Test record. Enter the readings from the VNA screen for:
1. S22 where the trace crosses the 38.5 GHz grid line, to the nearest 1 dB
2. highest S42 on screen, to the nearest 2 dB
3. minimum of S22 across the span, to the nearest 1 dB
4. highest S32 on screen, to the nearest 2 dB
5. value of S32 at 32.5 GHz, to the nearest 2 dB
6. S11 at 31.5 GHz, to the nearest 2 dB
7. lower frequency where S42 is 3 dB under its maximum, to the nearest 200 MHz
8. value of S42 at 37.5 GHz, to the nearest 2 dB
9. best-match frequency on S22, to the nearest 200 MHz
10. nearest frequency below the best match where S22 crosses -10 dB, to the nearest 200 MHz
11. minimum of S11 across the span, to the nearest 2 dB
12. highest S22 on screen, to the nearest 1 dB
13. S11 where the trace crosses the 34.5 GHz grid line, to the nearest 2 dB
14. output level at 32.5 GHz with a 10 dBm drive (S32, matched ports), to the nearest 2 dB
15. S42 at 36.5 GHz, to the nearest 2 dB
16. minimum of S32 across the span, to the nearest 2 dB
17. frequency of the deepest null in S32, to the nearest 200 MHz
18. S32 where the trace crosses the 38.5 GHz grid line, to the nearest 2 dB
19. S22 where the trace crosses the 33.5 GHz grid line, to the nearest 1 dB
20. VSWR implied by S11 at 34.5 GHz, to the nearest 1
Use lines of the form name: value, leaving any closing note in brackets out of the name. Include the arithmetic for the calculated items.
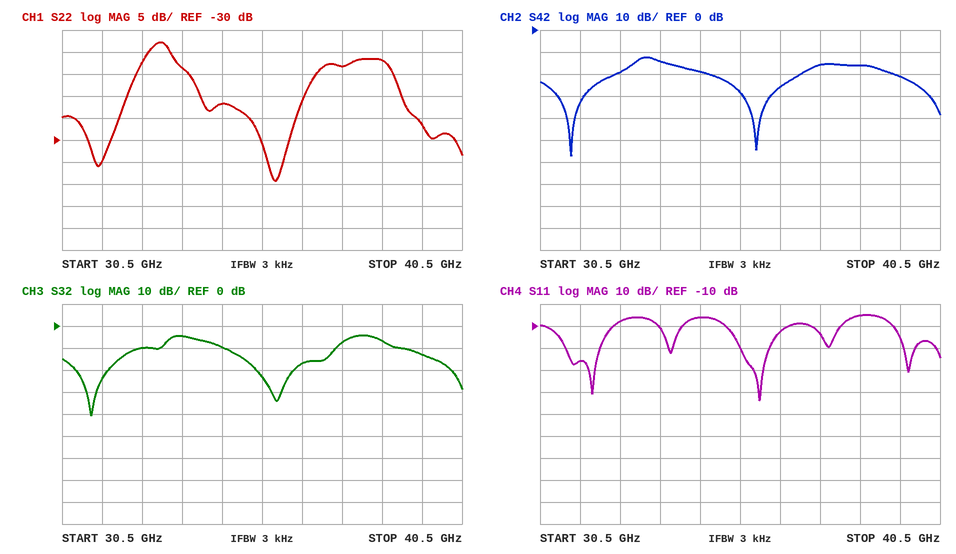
S22 where the trace crosses the 38.5 GHz grid line, to the nearest 1 dB: -12 dB
highest S42 on screen, to the nearest 2 dB: -12 dB
minimum of S22 across the span, to the nearest 1 dB: -39 dB
highest S32 on screen, to the nearest 2 dB: -4 dB
value of S32 at 32.5 GHz, to the nearest 2 dB: -10 dB
S11 at 31.5 GHz, to the nearest 2 dB: -26 dB
lower frequency where S42 is 3 dB under its maximum, to the nearest 200 MHz: 32.8 GHz
value of S42 at 37.5 GHz, to the nearest 2 dB: -16 dB
best-match frequency on S22, to the nearest 200 MHz: 35.8 GHz
nearest frequency below the best match where S22 crosses -10 dB, to the nearest 200 MHz: 33.2 GHz
minimum of S11 across the span, to the nearest 2 dB: -44 dB
highest S22 on screen, to the nearest 1 dB: -8 dB
S11 where the trace crosses the 34.5 GHz grid line, to the nearest 2 dB: -6 dB
output level at 32.5 GHz with a 10 dBm drive (S32, matched ports), to the nearest 2 dB: 10 dBm + (-10 dB) = 0 dBm
S42 at 36.5 GHz, to the nearest 2 dB: -26 dB
minimum of S32 across the span, to the nearest 2 dB: -40 dB
frequency of the deepest null in S32, to the nearest 200 MHz: 31.2 GHz
S32 where the trace crosses the 38.5 GHz grid line, to the nearest 2 dB: -6 dB
S22 where the trace crosses the 33.5 GHz grid line, to the nearest 1 dB: -14 dB
VSWR implied by S11 at 34.5 GHz, to the nearest 1: |Γ| = 10^(-6/20) = 0.5012; VSWR = (1 + 0.5012)/(1 − 0.5012) ≈ 3
